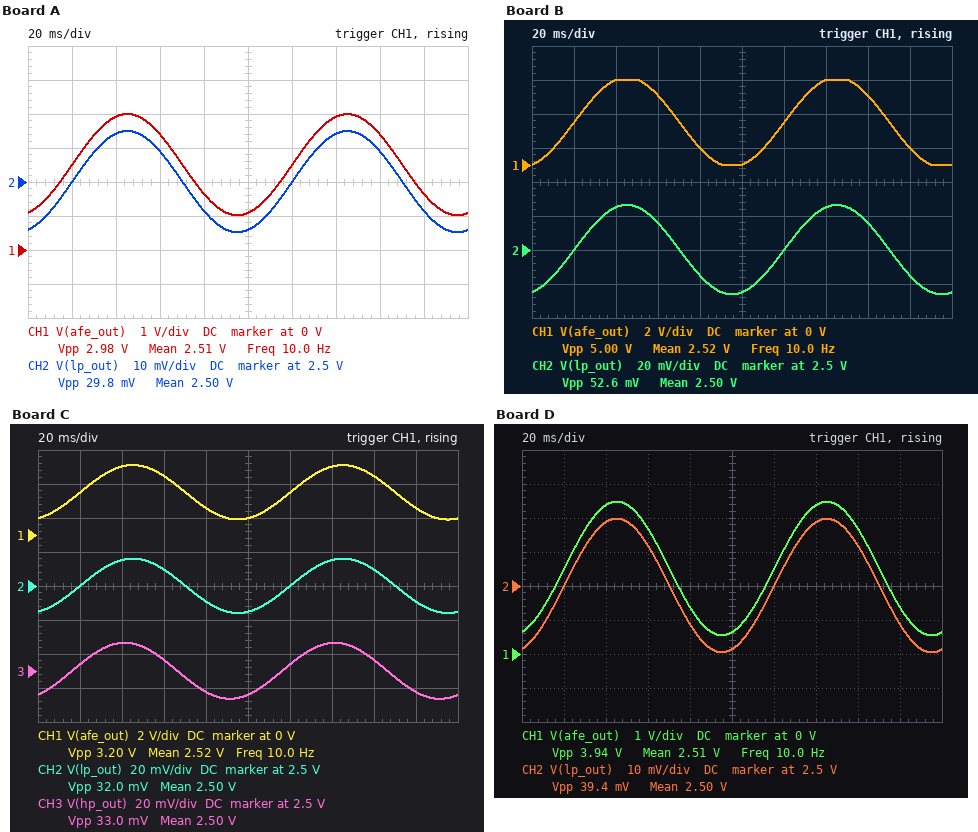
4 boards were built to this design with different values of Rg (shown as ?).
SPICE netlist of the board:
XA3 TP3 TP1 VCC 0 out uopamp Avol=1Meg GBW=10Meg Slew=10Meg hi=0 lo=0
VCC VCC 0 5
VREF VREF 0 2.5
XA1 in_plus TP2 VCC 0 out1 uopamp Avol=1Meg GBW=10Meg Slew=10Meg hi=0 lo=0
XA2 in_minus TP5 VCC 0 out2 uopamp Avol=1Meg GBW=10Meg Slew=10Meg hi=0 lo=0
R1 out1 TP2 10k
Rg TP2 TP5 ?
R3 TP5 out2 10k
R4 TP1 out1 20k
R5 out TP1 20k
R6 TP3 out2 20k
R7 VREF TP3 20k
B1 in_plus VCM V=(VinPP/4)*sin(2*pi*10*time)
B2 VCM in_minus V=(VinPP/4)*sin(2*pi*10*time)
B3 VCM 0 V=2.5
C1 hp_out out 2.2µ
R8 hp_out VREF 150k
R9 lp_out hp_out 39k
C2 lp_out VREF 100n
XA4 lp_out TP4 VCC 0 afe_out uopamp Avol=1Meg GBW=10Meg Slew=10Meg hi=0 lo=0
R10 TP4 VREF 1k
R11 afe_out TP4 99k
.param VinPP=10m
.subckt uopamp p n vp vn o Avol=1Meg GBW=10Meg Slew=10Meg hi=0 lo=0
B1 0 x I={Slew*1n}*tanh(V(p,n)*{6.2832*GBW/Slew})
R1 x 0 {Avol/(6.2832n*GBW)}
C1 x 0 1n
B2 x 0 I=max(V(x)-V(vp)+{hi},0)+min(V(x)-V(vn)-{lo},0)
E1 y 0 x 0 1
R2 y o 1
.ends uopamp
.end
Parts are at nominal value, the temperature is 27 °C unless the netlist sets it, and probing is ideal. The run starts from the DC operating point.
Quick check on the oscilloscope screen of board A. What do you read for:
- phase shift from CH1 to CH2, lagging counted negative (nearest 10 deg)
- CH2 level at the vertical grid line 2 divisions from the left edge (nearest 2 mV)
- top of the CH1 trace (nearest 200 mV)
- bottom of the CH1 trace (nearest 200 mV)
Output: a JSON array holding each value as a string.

["0 deg", "2.514 V", "4.0 V", "1.0 V"]
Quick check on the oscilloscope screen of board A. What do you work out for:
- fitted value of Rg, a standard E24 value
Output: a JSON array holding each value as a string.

["9.1 kΩ"]
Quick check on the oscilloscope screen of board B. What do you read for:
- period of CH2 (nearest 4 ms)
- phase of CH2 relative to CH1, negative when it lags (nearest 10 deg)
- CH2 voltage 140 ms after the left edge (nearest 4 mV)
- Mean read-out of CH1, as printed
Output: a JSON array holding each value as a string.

["100 ms", "0 deg", "2.524 V", "2.52 V"]
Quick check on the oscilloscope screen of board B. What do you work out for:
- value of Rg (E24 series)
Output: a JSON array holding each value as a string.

["4.3 kΩ"]
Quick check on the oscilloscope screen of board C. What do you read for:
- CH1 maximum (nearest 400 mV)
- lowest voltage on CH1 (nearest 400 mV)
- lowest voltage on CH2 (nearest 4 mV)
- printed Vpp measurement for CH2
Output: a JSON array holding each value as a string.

["4.0 V", "800 mV", "2.484 V", "32.0 mV"]
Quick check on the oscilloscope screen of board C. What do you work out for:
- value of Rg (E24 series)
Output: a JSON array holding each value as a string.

["8.2 kΩ"]
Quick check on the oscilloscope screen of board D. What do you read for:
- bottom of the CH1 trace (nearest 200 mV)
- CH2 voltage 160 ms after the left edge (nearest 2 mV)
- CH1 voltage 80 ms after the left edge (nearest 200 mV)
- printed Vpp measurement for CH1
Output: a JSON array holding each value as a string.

["600 mV", "2.512 V", "1.4 V", "3.94 V"]
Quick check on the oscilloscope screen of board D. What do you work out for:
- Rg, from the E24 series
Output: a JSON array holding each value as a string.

["6.2 kΩ"]
